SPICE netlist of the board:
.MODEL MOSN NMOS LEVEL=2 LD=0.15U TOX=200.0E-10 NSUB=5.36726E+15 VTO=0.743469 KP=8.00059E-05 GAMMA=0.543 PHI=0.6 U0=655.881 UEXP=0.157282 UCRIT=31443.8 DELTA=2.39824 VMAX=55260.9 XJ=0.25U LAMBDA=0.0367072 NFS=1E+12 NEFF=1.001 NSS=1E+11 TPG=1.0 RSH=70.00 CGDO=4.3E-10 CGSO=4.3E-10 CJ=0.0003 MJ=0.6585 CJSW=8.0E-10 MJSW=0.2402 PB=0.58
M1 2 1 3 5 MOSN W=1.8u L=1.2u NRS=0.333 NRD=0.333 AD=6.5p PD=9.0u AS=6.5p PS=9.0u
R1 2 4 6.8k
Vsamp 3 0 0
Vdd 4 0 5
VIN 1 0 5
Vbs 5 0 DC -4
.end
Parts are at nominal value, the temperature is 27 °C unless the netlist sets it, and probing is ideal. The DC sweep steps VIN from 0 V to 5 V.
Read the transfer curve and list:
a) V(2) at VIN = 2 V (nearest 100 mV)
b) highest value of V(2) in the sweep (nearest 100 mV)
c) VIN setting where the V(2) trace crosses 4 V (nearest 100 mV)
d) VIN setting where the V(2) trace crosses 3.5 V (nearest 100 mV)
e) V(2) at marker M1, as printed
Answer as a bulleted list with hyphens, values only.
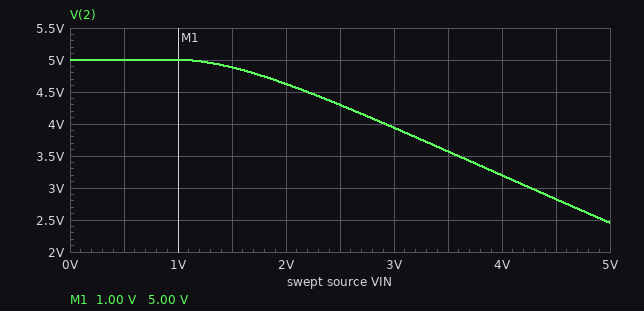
- 4.6 V
- 5.0 V
- 2.9 V
- 3.6 V
- 5.00 V
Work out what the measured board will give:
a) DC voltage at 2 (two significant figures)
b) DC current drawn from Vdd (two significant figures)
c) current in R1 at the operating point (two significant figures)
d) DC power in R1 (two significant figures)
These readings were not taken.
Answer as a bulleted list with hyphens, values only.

- 2.5 V
- 370 µA
- 370 µA
- 950 µW
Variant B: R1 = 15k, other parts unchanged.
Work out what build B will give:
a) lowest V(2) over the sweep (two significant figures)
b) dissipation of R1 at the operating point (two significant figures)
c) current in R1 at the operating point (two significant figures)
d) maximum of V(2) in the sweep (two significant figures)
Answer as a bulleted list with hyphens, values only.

- 800 mV
- 1.2 mW
- 280 µA
- 5.0 V
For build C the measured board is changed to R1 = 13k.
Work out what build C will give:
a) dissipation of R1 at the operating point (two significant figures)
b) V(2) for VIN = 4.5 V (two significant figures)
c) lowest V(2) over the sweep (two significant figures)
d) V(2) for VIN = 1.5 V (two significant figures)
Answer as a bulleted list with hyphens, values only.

- 1.3 mW
- 1.2 V
- 910 mV
- 4.8 V
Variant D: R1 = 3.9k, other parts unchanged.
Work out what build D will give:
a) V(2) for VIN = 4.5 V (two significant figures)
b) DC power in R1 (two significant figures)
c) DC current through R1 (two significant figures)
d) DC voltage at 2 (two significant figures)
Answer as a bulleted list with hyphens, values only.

- 3.7 V
- 600 µW
- 390 µA
- 3.5 V
